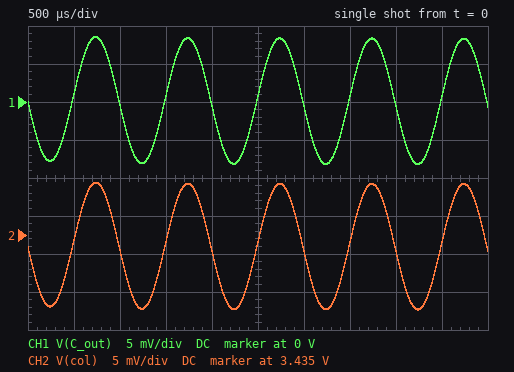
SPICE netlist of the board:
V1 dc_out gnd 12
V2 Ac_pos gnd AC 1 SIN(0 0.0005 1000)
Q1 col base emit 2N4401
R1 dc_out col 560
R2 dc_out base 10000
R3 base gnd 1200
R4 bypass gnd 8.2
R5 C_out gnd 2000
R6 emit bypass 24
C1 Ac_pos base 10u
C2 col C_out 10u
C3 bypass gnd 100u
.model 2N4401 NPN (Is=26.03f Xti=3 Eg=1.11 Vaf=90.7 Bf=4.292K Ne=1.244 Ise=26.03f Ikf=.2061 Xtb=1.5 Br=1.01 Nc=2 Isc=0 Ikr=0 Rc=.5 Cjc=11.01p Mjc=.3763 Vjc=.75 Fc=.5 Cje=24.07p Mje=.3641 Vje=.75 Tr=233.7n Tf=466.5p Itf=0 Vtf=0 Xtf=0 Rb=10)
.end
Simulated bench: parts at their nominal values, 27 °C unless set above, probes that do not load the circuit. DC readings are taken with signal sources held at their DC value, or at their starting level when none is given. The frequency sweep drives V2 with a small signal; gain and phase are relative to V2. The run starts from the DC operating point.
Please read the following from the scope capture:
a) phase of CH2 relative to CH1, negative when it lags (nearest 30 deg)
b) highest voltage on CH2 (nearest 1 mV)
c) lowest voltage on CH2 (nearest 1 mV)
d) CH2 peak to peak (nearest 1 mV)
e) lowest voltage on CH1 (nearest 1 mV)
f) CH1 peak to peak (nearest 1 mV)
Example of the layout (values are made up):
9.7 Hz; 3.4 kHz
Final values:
0 deg; 3.442 V; 3.425 V; 17 mV; -8 mV; 17 mV
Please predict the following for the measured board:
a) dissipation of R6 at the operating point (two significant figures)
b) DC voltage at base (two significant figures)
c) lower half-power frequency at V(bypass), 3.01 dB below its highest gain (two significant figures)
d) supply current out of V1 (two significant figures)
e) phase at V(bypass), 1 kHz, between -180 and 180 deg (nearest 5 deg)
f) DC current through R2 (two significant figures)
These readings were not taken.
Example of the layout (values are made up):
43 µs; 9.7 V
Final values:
5.7 mW; 1.2 V; 15 Hz; 16 mA; -75 deg; 1.1 mA
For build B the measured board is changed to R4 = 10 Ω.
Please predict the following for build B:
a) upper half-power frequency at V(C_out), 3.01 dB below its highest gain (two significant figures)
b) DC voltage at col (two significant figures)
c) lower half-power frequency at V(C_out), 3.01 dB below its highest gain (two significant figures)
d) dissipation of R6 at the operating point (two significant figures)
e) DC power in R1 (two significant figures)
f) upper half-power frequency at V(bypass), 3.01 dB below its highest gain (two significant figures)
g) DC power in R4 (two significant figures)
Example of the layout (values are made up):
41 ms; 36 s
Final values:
39 MHz; 3.8 V; 58 Hz; 5.2 mW; 120 mW; 250 Hz; 2.2 mW
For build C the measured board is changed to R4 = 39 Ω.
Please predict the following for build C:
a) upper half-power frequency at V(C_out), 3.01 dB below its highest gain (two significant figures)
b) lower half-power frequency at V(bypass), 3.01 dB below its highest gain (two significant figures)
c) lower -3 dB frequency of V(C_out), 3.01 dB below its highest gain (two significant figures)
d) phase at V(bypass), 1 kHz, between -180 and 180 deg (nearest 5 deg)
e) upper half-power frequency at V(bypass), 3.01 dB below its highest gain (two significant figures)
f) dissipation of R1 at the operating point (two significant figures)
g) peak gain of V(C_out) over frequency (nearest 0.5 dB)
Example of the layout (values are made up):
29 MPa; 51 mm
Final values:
50 MHz; 12 Hz; 87 Hz; -85 deg; 130 Hz; 42 mW; 24.0 dB
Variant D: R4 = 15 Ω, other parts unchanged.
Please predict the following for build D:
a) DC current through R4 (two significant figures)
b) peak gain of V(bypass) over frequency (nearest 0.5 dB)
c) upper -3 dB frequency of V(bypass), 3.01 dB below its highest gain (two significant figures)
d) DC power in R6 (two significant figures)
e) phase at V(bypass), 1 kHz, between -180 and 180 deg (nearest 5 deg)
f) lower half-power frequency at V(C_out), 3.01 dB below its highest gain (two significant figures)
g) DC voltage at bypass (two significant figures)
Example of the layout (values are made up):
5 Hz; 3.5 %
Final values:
13 mA; -9.5 dB; 200 Hz; 4.1 mW; -80 deg; 85 Hz; 200 mV
